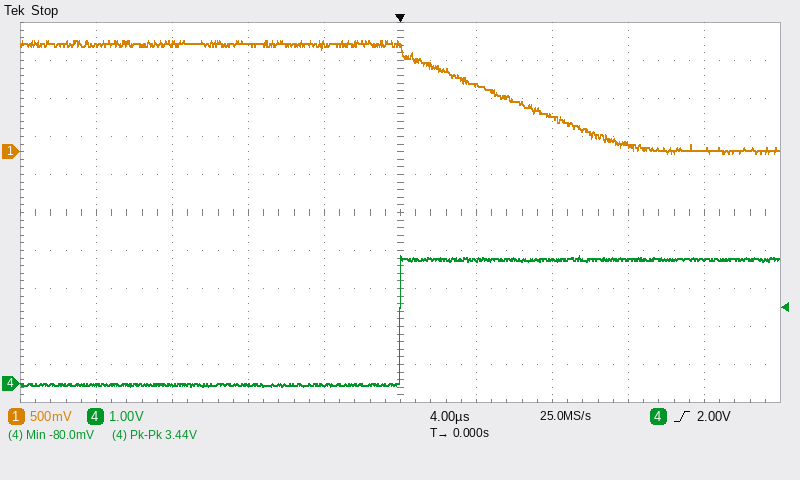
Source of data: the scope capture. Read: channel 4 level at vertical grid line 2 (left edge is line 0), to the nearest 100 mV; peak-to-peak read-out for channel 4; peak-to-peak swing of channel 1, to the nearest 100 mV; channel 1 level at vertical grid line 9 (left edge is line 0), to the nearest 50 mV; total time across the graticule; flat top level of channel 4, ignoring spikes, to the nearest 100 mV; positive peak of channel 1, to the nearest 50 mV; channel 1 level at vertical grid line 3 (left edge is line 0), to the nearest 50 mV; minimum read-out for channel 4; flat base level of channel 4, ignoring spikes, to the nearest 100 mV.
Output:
0.0 V
3.44 V
1.50 V
50 mV
40 µs
3.3 V
1.45 V
1.40 V
-80.0 mV
0.0 V
